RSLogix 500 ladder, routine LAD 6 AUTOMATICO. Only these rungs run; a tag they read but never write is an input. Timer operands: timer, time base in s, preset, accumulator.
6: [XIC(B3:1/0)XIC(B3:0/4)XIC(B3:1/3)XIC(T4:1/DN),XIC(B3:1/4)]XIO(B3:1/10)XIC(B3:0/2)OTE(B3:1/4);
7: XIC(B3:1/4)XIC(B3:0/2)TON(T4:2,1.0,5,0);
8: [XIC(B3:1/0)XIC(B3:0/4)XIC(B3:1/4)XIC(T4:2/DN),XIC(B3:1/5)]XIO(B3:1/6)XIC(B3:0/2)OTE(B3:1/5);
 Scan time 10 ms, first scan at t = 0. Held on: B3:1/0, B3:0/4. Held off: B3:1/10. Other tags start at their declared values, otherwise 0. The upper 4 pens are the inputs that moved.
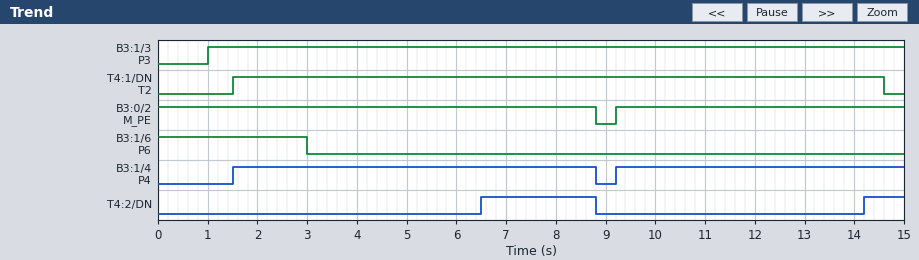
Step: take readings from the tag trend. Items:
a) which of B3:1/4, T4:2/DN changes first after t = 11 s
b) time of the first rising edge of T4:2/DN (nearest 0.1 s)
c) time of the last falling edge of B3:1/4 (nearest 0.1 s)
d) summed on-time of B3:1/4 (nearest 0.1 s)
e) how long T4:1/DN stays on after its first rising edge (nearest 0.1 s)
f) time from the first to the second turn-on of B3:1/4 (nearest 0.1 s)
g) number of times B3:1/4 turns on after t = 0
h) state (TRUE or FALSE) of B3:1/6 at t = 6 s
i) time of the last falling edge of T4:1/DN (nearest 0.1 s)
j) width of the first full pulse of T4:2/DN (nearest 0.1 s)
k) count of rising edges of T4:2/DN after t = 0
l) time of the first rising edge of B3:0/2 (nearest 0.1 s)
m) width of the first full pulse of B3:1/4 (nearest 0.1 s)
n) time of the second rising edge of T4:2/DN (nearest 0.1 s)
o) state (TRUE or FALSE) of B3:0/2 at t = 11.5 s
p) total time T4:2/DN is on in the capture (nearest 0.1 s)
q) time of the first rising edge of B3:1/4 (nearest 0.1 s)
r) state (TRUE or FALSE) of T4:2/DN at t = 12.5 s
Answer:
T4:2/DN
6.5 s
8.8 s
13.1 s
13.1 s
7.7 s
2
FALSE
14.6 s
2.3 s
2
9.2 s
7.3 s
14.2 s
TRUE
3.1 s
1.5 s
FALSE
